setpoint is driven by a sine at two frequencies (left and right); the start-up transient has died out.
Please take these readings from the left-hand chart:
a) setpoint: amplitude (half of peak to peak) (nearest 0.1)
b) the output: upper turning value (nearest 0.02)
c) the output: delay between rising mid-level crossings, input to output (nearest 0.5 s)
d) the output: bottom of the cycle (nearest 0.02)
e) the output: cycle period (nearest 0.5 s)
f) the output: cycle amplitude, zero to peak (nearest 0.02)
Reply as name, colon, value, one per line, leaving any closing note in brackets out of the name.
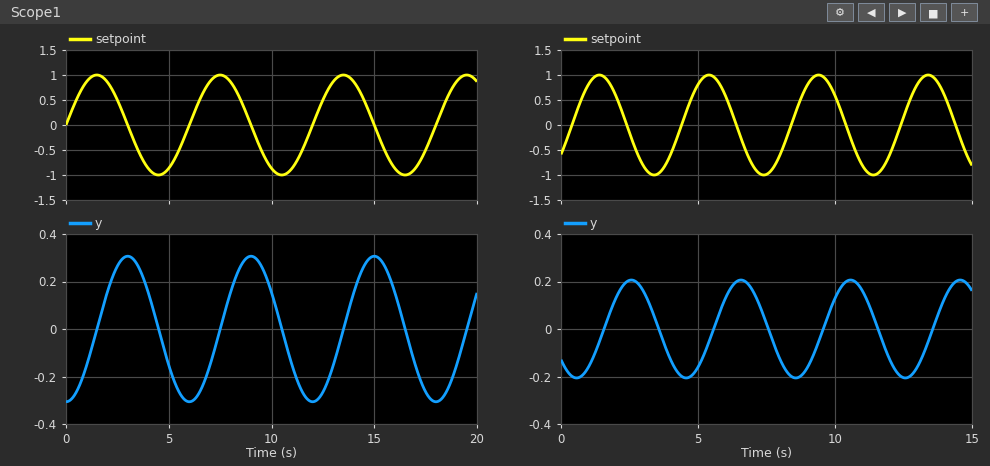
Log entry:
setpoint: amplitude (half of peak to peak): 1.0
the output: upper turning value: 0.30
the output: delay between rising mid-level crossings, input to output: 1.5 s
the output: bottom of the cycle: -0.30
the output: cycle period: 6.0 s
the output: cycle amplitude, zero to peak: 0.30
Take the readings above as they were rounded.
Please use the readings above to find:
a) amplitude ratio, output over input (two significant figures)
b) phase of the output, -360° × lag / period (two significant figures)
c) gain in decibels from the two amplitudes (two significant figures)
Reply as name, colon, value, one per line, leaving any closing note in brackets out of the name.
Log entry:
amplitude ratio, output over input: 0.30
phase of the output, -360° × lag / period: -90°
gain in decibels from the two amplitudes: -10 dB
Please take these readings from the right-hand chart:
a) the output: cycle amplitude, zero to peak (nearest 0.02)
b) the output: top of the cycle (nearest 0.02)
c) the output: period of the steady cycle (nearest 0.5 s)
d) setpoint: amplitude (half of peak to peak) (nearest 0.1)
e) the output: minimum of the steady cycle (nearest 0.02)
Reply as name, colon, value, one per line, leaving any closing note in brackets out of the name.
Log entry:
the output: cycle amplitude, zero to peak: 0.20
the output: top of the cycle: 0.20
the output: period of the steady cycle: 4.0 s
setpoint: amplitude (half of peak to peak): 1.0
the output: minimum of the steady cycle: -0.20
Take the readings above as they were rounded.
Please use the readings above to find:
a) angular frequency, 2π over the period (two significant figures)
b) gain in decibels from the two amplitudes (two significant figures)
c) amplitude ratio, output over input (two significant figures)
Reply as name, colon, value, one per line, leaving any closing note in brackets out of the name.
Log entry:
angular frequency, 2π over the period: 1.6 rad/s
gain in decibels from the two amplitudes: -14 dB
amplitude ratio, output over input: 0.20
